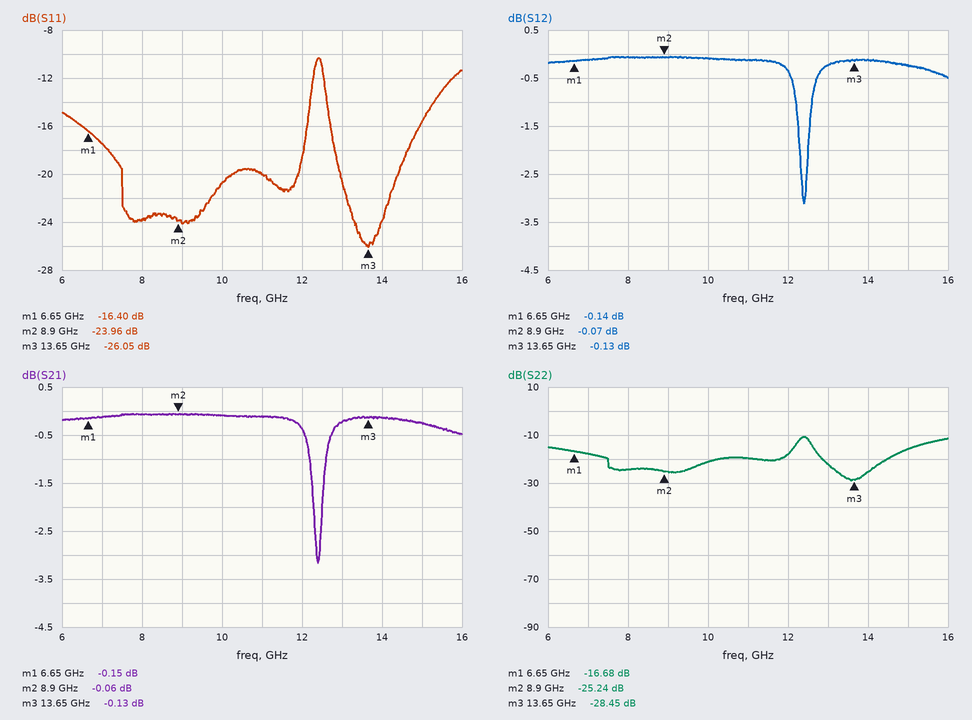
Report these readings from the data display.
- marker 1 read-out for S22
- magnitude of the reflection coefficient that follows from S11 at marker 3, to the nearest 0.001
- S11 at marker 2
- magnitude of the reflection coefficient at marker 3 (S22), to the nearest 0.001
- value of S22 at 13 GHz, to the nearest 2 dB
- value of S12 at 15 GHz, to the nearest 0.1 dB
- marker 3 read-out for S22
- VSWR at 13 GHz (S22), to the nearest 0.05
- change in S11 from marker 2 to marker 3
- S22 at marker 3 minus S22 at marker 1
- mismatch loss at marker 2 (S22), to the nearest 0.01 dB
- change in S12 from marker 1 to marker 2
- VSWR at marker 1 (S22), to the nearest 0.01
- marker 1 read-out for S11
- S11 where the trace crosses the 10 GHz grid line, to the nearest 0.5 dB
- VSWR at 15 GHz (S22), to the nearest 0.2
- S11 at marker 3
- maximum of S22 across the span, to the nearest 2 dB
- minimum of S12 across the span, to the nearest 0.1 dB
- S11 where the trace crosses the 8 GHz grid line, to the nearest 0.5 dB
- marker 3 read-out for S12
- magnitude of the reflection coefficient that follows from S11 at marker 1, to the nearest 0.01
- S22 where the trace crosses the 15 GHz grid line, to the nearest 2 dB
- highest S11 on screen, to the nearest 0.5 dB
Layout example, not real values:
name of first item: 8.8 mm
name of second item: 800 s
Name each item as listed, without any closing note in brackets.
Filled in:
marker 1 read-out for S22: -16.68 dB
magnitude of the reflection coefficient that follows from S11 at marker 3, to the nearest 0.001: 0.050
S11 at marker 2: -23.96 dB
magnitude of the reflection coefficient at marker 3 (S22), to the nearest 0.001: 0.038
value of S22 at 13 GHz, to the nearest 2 dB: -22 dB
value of S12 at 15 GHz, to the nearest 0.1 dB: -0.2 dB
marker 3 read-out for S22: -28.45 dB
VSWR at 13 GHz (S22), to the nearest 0.05: 1.15
change in S11 from marker 2 to marker 3: -2.09 dB
S22 at marker 3 minus S22 at marker 1: -11.77 dB
mismatch loss at marker 2 (S22), to the nearest 0.01 dB: 0.01 dB
change in S12 from marker 1 to marker 2: 0.07 dB
VSWR at marker 1 (S22), to the nearest 0.01: 1.34
marker 1 read-out for S11: -16.40 dB
S11 where the trace crosses the 10 GHz grid line, to the nearest 0.5 dB: -20.5 dB
VSWR at 15 GHz (S22), to the nearest 0.2: 1.4
S11 at marker 3: -26.05 dB
maximum of S22 across the span, to the nearest 2 dB: -10 dB
minimum of S12 across the span, to the nearest 0.1 dB: -3.1 dB
S11 where the trace crosses the 8 GHz grid line, to the nearest 0.5 dB: -24.0 dB
marker 3 read-out for S12: -0.13 dB
magnitude of the reflection coefficient that follows from S11 at marker 1, to the nearest 0.01: 0.15
S22 where the trace crosses the 15 GHz grid line, to the nearest 2 dB: -16 dB
highest S11 on screen, to the nearest 0.5 dB: -10.5 dB
